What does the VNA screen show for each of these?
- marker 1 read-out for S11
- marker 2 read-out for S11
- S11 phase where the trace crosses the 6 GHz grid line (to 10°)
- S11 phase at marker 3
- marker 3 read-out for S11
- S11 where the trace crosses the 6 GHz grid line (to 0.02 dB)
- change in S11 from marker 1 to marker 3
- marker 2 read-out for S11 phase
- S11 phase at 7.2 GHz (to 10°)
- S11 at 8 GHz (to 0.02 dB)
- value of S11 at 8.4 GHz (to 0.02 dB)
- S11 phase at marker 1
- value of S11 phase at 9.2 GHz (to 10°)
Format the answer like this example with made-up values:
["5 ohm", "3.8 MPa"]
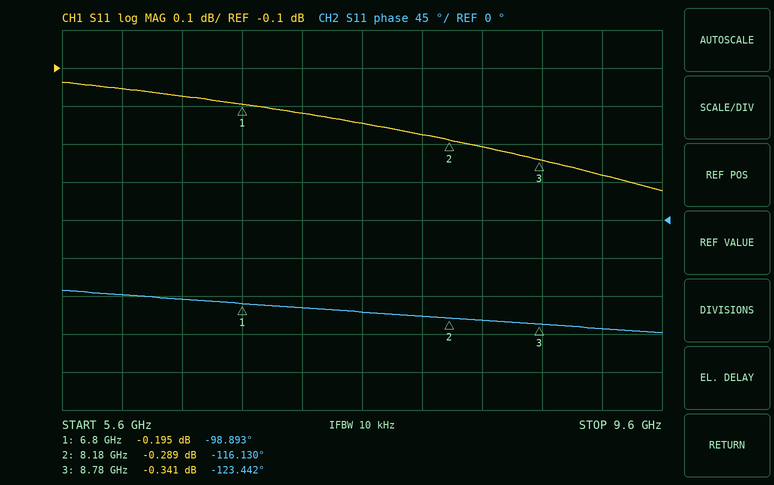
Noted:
["-0.195 dB", "-0.289 dB", "-90°", "-123.442°", "-0.341 dB", "-0.16 dB", "-0.146 dB", "-116.130°", "-100°", "-0.28 dB", "-0.30 dB", "-98.893°", "-130°"]
